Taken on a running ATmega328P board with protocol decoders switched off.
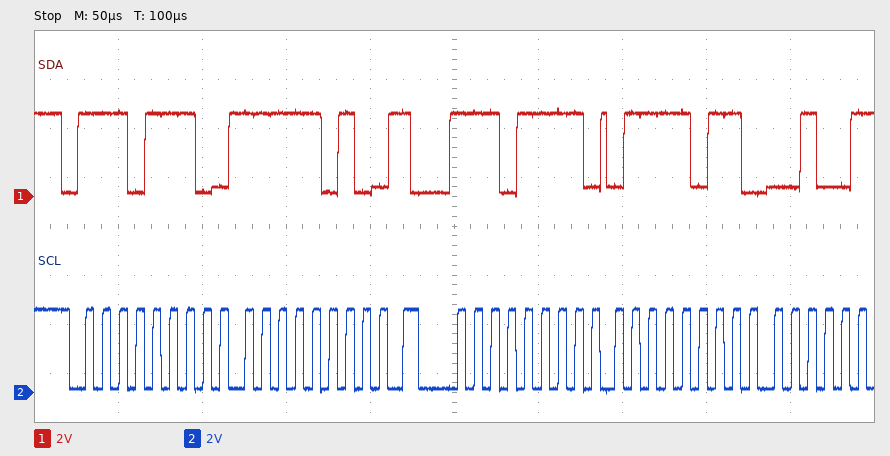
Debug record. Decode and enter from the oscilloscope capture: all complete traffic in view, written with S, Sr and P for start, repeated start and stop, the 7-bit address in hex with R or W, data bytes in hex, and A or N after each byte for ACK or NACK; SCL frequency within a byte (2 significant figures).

S 77W A FA A Sr 77R A 7B A
100 kHz
